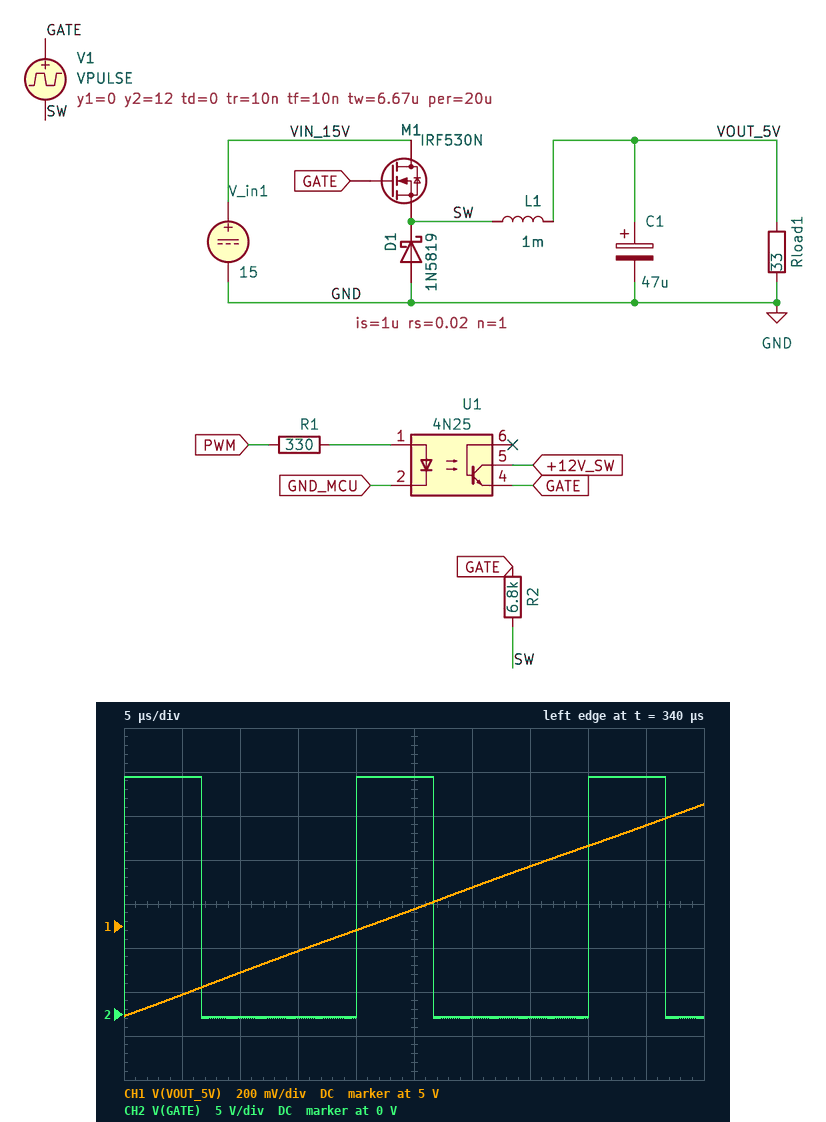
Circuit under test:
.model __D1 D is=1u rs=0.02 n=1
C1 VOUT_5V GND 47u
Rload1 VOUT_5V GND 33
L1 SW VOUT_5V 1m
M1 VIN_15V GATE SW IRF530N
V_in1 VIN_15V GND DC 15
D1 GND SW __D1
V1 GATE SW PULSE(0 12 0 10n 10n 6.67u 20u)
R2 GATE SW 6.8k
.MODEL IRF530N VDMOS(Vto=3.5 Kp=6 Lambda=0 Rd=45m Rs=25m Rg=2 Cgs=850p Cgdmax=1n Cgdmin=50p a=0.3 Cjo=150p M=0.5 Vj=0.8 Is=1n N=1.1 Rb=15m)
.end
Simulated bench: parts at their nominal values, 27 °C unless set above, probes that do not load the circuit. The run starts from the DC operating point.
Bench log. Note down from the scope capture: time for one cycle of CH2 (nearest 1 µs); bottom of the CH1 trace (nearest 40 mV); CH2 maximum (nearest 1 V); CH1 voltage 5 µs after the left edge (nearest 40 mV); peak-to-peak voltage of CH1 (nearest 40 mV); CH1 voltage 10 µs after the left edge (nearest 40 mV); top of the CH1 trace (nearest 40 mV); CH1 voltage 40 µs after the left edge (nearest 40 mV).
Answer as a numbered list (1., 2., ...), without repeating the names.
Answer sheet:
1. 20 µs
2. 4.60 V
3. 27 V
4. 4.68 V
5. 960 mV
6. 4.80 V
7. 5.56 V
8. 5.36 V
